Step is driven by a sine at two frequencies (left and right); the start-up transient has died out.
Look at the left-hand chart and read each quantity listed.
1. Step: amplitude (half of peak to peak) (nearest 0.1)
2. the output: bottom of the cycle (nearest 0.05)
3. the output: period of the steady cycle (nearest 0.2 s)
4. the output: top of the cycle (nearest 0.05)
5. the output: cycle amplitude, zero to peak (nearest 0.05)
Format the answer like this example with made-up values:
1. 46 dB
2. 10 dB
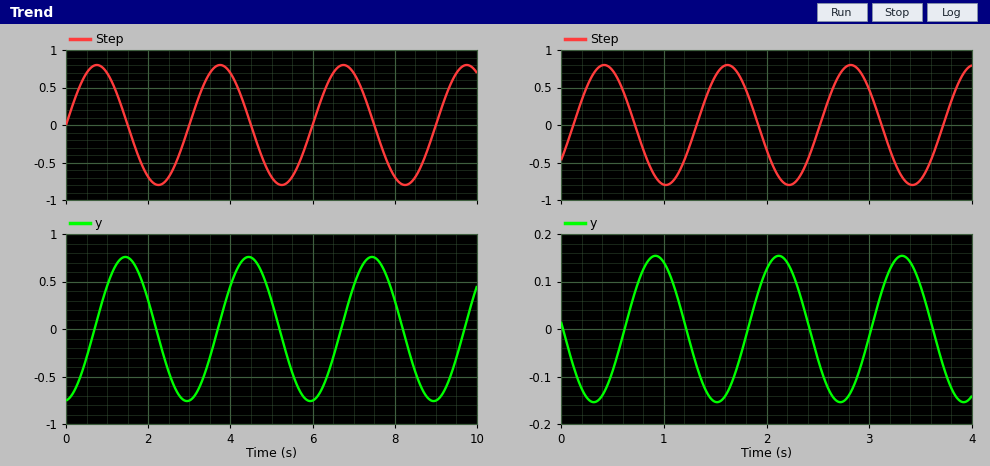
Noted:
1. 0.8
2. -0.75
3. 3.0 s
4. 0.75
5. 0.75
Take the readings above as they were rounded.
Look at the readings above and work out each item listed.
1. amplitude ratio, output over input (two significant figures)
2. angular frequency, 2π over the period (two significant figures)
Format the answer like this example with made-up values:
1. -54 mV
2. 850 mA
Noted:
1. 0.94
2. 2.1 rad/s
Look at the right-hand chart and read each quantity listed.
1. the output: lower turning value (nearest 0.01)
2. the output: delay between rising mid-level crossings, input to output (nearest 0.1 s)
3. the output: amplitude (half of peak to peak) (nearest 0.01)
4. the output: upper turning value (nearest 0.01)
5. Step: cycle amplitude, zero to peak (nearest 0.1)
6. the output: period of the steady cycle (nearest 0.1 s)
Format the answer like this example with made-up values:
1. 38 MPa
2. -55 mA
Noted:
1. -0.15
2. 0.5 s
3. 0.15
4. 0.15
5. 0.8
6. 1.2 s
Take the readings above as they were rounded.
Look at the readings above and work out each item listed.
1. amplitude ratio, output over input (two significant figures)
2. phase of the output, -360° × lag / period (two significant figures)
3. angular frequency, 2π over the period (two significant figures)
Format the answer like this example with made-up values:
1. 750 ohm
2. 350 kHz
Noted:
1. 0.19
2. -150°
3. 5.2 rad/s
